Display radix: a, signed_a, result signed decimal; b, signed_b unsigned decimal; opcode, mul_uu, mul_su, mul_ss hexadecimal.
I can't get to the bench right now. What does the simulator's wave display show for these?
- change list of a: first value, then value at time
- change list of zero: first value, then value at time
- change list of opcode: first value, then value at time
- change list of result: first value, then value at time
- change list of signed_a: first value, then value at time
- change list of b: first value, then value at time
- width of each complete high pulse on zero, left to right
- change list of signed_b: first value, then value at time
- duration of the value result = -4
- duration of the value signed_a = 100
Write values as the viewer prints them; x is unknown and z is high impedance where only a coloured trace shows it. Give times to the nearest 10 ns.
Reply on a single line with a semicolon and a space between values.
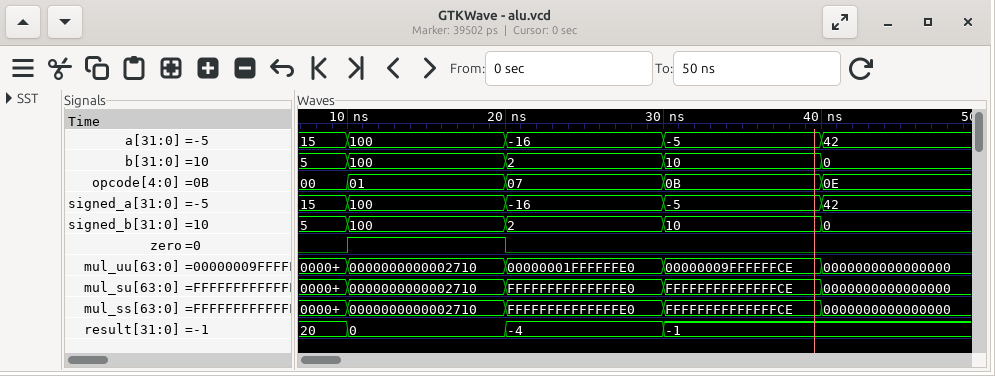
15, 100 at 10 ns, -16 at 20 ns, -5 at 30 ns, 42 at 40 ns; 0, 1 at 10 ns, 0 at 20 ns; 00, 01 at 10 ns, 07 at 20 ns, 0B at 30 ns, 0E at 40 ns; 20, 0 at 10 ns, -4 at 20 ns, -1 at 30 ns; 15, 100 at 10 ns, -16 at 20 ns, -5 at 30 ns, 42 at 40 ns; 5, 100 at 10 ns, 2 at 20 ns, 10 at 30 ns, 0 at 40 ns; 10 ns; 5, 100 at 10 ns, 2 at 20 ns, 10 at 30 ns, 0 at 40 ns; 10 ns; 10 ns
